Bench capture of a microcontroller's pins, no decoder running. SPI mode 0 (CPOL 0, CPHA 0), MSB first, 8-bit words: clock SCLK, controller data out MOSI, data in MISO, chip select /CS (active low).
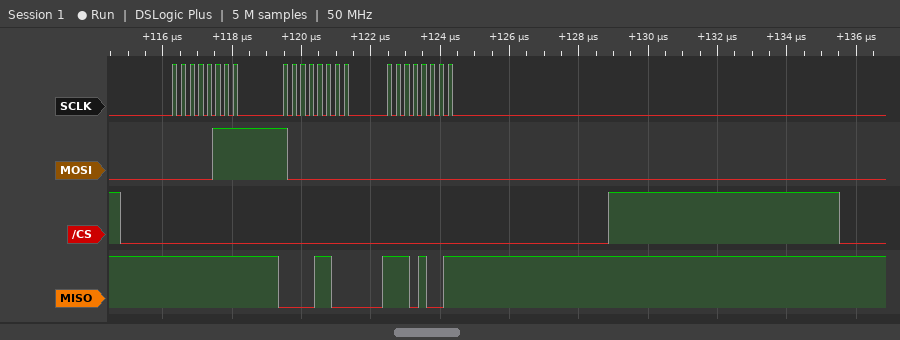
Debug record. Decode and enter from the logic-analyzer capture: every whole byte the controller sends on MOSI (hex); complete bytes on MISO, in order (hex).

07 80 00
FF 0C E9
